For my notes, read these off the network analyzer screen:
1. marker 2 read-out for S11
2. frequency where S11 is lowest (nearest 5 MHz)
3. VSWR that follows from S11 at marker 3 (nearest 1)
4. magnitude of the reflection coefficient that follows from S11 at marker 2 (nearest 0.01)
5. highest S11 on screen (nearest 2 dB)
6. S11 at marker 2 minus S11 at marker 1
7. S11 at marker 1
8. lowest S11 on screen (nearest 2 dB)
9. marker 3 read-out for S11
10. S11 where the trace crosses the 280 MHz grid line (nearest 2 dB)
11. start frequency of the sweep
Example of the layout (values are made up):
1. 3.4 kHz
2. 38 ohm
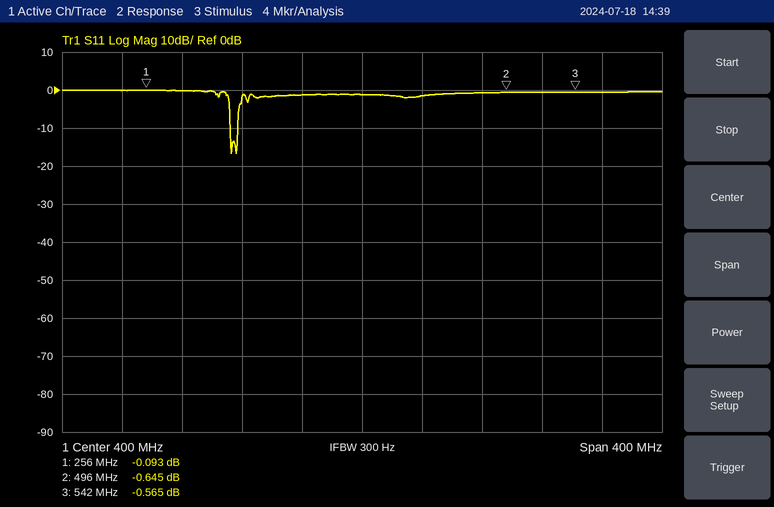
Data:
1. -0.645 dB
2. 315 MHz
3. 31
4. 0.93
5. 0 dB
6. -0.552 dB
7. -0.093 dB
8. -16 dB
9. -0.565 dB
10. 0 dB
11. 200 MHz
